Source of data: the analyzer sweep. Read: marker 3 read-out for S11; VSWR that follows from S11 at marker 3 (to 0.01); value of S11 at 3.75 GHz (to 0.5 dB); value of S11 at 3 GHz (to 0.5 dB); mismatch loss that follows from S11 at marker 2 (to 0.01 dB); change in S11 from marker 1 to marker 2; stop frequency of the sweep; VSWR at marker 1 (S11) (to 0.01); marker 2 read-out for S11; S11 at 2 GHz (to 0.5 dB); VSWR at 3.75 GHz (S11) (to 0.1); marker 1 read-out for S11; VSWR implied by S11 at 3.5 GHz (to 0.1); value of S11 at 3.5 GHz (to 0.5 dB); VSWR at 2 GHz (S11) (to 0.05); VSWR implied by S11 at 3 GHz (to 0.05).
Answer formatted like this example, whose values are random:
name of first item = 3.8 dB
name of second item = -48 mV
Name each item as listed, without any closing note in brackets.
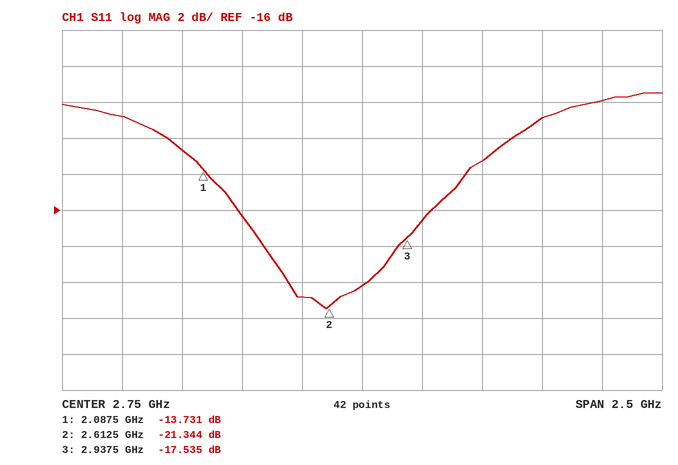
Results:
marker 3 read-out for S11 = -17.535 dB
VSWR that follows from S11 at marker 3 = 1.31
value of S11 at 3.75 GHz = -10.0 dB
value of S11 at 3 GHz = -16.5 dB
mismatch loss that follows from S11 at marker 2 = 0.03 dB
change in S11 from marker 1 to marker 2 = -7.613 dB
stop frequency of the sweep = 4 GHz
VSWR at marker 1 (S11) = 1.52
marker 2 read-out for S11 = -21.344 dB
S11 at 2 GHz = -12.5 dB
VSWR at 3.75 GHz (S11) = 1.9
marker 1 read-out for S11 = -13.731 dB
VSWR implied by S11 at 3.5 GHz = 1.8
value of S11 at 3.5 GHz = -11.0 dB
VSWR at 2 GHz (S11) = 1.60
VSWR implied by S11 at 3 GHz = 1.35
